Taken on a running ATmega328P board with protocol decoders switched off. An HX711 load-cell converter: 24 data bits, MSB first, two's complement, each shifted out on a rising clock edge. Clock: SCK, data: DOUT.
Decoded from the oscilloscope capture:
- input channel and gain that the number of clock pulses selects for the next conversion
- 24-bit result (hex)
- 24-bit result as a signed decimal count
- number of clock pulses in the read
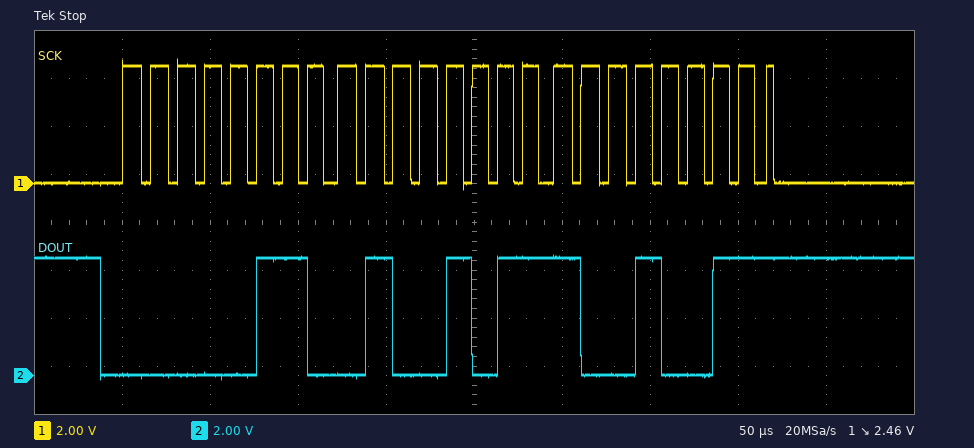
channel A, gain 128
0x064B93
412563
25
